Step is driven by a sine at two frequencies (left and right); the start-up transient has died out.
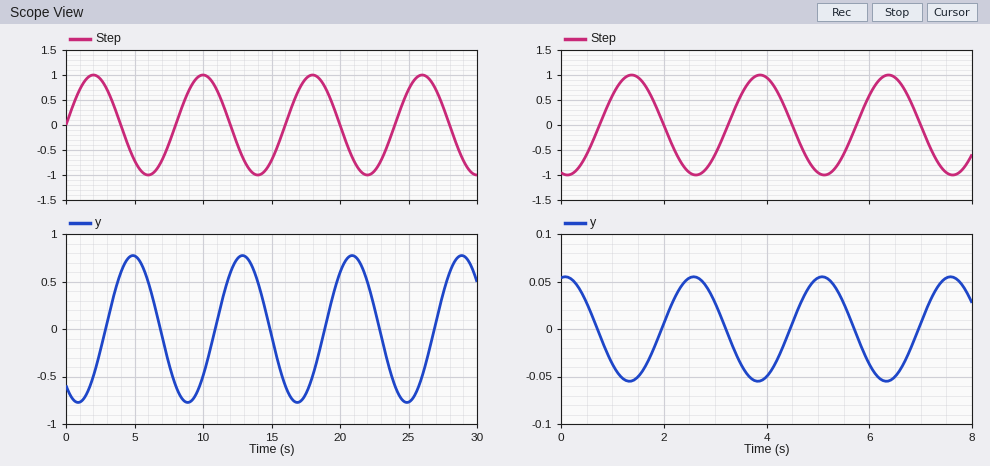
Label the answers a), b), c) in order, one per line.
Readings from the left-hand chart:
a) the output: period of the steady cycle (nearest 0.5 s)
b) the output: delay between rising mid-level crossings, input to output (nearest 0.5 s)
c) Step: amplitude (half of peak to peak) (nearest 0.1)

a) 8.0 s
b) 3.0 s
c) 1.0
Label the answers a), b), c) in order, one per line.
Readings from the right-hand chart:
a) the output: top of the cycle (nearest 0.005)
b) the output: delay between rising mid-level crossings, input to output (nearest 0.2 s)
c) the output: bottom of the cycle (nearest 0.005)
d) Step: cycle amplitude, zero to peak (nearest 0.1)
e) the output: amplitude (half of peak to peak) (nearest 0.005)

a) 0.055
b) 1.2 s
c) -0.055
d) 1.0
e) 0.055
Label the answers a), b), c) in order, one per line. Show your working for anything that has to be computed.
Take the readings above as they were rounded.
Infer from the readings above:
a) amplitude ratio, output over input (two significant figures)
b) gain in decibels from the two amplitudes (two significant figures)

a) 0.055 / 1 = 0.055
b) 20 log10(0.055 / 1) = -25 dB
